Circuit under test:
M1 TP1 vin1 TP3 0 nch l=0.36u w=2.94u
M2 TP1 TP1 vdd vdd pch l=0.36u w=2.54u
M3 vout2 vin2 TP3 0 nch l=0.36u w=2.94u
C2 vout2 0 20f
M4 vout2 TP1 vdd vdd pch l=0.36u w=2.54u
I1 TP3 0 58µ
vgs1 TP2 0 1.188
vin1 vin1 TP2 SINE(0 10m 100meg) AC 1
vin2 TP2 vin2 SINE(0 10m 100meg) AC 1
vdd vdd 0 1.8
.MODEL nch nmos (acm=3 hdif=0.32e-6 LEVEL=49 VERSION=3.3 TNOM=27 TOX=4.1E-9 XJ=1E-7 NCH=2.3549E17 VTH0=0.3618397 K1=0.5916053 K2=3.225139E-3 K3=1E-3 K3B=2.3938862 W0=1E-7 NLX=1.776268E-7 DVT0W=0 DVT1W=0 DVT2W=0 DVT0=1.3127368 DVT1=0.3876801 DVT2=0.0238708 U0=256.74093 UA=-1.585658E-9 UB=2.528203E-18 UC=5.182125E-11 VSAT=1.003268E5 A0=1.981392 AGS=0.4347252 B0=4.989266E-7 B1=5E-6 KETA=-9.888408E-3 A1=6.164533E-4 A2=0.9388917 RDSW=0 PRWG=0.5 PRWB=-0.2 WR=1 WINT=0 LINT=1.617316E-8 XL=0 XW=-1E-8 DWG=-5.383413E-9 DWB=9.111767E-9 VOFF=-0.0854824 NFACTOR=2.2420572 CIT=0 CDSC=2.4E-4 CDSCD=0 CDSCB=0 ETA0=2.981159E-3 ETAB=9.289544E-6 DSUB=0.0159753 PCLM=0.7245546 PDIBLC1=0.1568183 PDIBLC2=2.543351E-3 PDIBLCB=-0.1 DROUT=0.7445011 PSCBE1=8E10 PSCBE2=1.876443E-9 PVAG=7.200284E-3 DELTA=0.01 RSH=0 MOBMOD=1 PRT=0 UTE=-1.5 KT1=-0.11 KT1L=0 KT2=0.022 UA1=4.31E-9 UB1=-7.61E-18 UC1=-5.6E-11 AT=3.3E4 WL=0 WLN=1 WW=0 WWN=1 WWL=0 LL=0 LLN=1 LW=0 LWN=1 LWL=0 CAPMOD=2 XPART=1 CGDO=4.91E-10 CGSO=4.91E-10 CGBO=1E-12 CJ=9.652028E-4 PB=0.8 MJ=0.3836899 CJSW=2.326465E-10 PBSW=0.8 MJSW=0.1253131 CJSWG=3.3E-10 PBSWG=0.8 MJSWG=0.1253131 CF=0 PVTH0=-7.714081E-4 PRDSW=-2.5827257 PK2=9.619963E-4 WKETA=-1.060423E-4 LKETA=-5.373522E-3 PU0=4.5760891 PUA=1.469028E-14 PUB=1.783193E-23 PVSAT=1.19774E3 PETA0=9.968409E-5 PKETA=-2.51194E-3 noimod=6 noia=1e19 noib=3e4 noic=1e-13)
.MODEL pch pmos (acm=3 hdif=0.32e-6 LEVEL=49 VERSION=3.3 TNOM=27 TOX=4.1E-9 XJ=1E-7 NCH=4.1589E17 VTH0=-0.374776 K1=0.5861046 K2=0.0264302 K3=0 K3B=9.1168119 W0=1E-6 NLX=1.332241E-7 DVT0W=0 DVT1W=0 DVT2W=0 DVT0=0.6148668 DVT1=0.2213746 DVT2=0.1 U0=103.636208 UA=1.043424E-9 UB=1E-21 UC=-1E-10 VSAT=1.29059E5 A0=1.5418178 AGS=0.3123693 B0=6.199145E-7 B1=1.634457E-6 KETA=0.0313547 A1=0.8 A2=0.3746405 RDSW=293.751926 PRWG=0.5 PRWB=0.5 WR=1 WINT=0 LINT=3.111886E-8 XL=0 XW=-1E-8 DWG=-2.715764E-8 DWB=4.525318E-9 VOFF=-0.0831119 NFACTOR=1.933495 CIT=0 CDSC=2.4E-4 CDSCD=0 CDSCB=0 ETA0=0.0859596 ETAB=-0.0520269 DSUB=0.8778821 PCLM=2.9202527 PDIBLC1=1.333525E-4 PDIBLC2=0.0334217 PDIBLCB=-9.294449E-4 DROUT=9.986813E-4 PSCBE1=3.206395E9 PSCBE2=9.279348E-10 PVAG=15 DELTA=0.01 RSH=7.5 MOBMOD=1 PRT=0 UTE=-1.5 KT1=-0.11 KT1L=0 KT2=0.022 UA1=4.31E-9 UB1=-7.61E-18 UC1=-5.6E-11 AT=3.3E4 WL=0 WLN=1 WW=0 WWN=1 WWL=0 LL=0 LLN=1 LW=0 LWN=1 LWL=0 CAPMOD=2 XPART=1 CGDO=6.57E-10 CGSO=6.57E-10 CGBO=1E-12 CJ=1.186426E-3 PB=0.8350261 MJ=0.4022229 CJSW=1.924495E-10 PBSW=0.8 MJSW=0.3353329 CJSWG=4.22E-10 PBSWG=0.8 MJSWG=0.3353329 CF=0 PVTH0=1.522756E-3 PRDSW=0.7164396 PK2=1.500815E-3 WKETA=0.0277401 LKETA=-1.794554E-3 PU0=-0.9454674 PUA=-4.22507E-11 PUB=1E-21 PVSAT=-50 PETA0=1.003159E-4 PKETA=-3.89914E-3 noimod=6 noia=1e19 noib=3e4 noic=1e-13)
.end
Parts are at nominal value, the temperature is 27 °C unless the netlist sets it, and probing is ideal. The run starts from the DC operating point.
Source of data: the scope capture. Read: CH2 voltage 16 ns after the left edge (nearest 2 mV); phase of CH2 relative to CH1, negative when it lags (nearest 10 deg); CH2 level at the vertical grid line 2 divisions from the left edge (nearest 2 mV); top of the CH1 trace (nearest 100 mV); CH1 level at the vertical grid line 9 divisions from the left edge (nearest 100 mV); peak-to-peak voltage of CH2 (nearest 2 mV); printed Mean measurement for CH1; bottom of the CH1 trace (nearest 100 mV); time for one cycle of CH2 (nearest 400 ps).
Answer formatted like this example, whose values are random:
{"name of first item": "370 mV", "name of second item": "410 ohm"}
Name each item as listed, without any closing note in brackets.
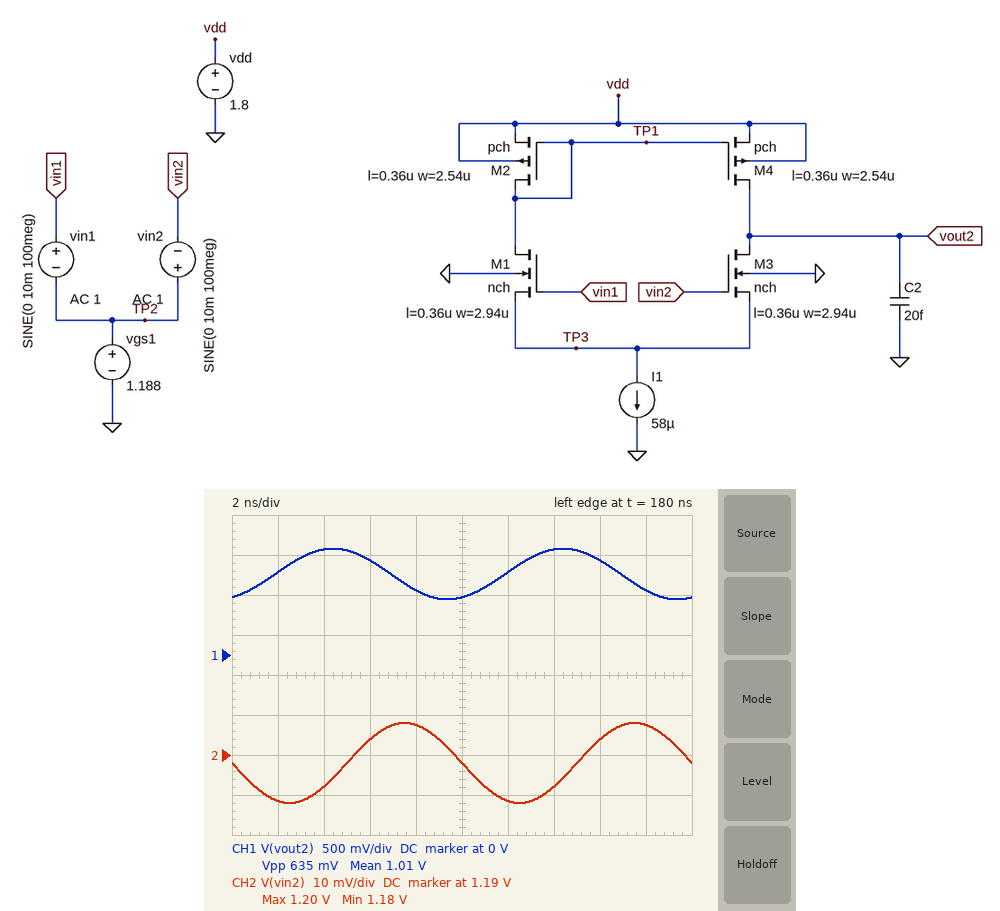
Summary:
{"CH2 voltage 16 ns after the left edge": "1.194 V", "phase of CH2 relative to CH1, negative when it lags": "-110 deg", "CH2 level at the vertical grid line 2 divisions from the left edge": "1.182 V", "top of the CH1 trace": "1.3 V", "CH1 level at the vertical grid line 9 divisions from the left edge": "800 mV", "peak-to-peak voltage of CH2": "20 mV", "printed Mean measurement for CH1": "1.01 V", "bottom of the CH1 trace": "700 mV", "time for one cycle of CH2": "10.0 ns"}
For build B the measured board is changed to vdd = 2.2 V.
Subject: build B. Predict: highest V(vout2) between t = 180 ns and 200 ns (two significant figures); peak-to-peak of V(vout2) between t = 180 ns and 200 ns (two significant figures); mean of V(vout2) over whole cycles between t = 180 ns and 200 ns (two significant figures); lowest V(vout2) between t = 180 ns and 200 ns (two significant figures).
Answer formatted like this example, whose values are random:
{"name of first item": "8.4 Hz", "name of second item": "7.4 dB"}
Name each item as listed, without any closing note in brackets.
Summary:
{"highest V(vout2) between t = 180 ns and 200 ns": "1.7 V", "peak-to-peak of V(vout2) between t = 180 ns and 200 ns": "650 mV", "mean of V(vout2) over whole cycles between t = 180 ns and 200 ns": "1.4 V", "lowest V(vout2) between t = 180 ns and 200 ns": "1.1 V"}
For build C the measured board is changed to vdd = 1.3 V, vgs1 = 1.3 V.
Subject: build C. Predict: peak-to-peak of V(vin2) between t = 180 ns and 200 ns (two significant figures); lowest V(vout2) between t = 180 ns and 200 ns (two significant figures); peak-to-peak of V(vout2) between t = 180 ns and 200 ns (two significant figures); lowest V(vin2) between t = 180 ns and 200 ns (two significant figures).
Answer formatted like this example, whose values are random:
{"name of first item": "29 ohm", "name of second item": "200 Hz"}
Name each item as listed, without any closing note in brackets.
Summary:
{"peak-to-peak of V(vin2) between t = 180 ns and 200 ns": "20 mV", "lowest V(vout2) between t = 180 ns and 200 ns": "500 mV", "peak-to-peak of V(vout2) between t = 180 ns and 200 ns": "12 mV", "lowest V(vin2) between t = 180 ns and 200 ns": "1.3 V"}
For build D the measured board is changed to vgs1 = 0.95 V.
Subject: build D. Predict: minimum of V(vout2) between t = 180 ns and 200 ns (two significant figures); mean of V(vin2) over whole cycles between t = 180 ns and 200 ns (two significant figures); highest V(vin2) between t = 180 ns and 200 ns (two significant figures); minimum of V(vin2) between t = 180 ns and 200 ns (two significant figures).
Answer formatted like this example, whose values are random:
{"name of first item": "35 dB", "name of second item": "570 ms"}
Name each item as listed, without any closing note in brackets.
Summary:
{"minimum of V(vout2) between t = 180 ns and 200 ns": "680 mV", "mean of V(vin2) over whole cycles between t = 180 ns and 200 ns": "950 mV", "highest V(vin2) between t = 180 ns and 200 ns": "960 mV", "minimum of V(vin2) between t = 180 ns and 200 ns": "940 mV"}
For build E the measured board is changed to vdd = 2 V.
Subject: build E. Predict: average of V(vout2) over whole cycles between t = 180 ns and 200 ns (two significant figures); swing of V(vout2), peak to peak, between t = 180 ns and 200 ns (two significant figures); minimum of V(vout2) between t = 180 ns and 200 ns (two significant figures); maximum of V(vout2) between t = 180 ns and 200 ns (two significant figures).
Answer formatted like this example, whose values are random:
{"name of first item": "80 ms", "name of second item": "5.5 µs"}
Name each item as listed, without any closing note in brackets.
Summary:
{"average of V(vout2) over whole cycles between t = 180 ns and 200 ns": "1.2 V", "swing of V(vout2), peak to peak, between t = 180 ns and 200 ns": "650 mV", "minimum of V(vout2) between t = 180 ns and 200 ns": "880 mV", "maximum of V(vout2) between t = 180 ns and 200 ns": "1.5 V"}
